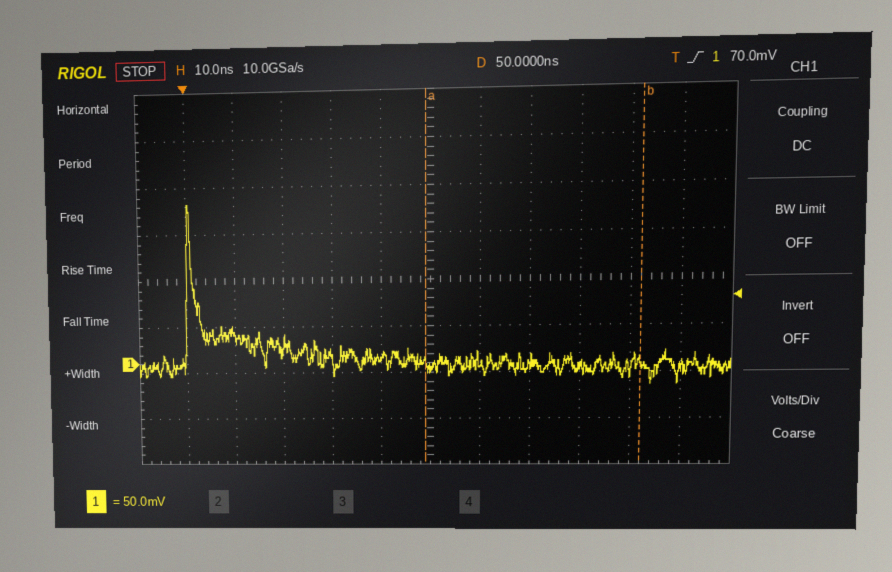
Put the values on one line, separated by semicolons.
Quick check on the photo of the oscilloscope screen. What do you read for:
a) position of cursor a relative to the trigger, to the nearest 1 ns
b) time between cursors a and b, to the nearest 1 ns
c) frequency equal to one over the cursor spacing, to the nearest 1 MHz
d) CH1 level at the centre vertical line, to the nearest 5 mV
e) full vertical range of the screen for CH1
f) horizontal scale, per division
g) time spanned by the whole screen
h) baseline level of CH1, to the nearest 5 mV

+49 ns; 43 ns; 23 MHz; -5 mV; 400 mV; 10 ns; 120 ns; 0 mV
